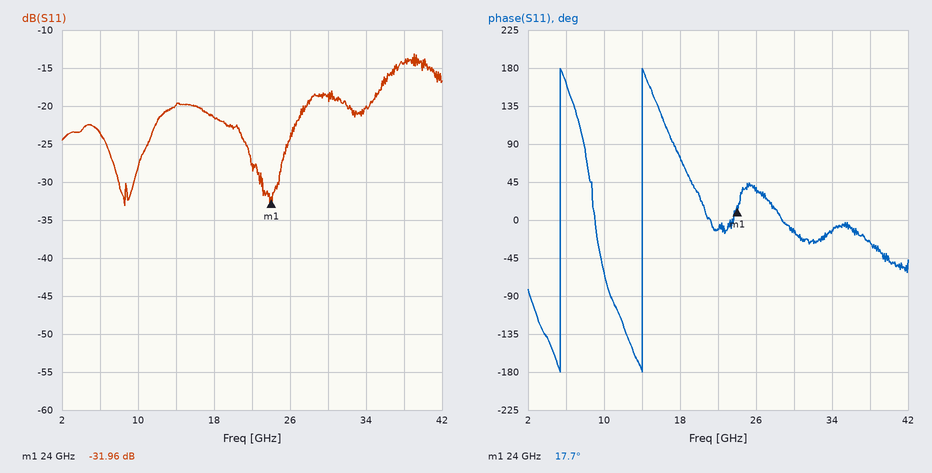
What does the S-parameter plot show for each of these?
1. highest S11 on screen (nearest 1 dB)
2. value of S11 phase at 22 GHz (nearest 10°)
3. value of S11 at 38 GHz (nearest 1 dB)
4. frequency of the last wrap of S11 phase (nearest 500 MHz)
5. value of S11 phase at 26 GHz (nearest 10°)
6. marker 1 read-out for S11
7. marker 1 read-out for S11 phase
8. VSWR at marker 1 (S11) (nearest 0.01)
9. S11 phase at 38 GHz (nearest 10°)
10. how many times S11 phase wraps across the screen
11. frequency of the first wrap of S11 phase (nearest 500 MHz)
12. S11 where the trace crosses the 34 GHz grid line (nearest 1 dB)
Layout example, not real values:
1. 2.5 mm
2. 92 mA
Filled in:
1. -13 dB
2. -10°
3. -14 dB
4. 14.0 GHz
5. 40°
6. -31.96 dB
7. 17.7°
8. 1.05
9. -30°
10. 2
11. 5.5 GHz
12. -20 dB
